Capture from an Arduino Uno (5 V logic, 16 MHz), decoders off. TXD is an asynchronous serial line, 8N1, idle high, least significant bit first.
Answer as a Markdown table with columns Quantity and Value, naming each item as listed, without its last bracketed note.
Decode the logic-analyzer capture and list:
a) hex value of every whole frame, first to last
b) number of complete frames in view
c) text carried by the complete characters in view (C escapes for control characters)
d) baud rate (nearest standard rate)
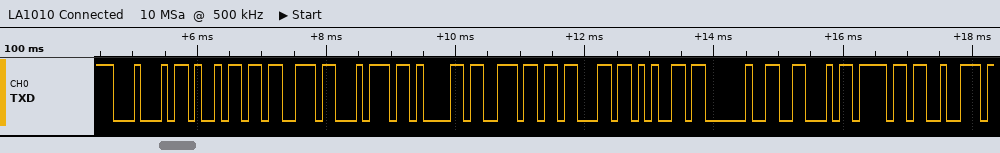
| Quantity | Value |
|---|---|
| hex value of every whole frame, first to last | 0x44 0x69 0x73 0x74 0x61 0x6E 0x63 0x65 0x20 0x46 0x6F 0x72 |
| number of complete frames in view | 12 |
| text carried by the complete characters in view | "Distance For" |
| baud rate | 9600 baud |
